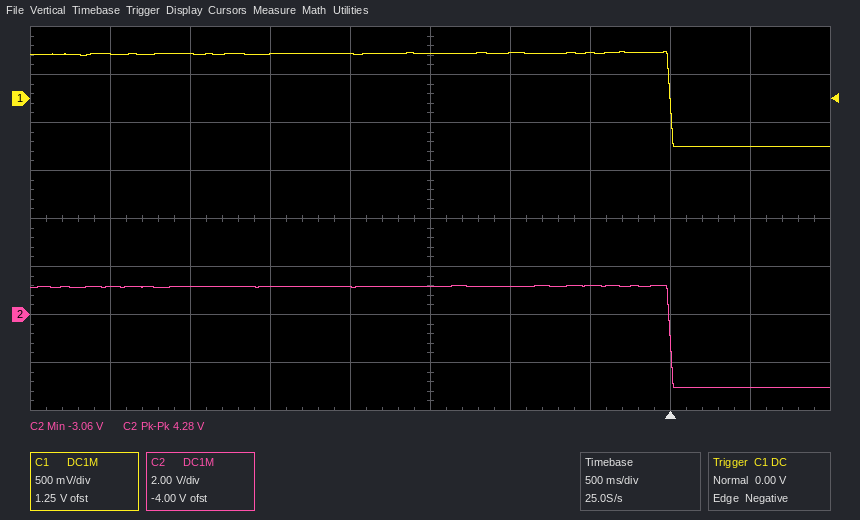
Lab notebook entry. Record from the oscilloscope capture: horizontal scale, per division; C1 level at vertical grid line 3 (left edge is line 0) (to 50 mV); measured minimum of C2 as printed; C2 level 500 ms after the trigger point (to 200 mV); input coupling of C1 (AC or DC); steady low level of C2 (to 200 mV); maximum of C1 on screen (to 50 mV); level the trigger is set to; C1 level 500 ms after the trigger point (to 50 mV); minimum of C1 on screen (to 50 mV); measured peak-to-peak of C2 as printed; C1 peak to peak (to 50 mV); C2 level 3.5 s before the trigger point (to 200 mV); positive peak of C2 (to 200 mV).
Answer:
500 ms
450 mV
-3.06 V
-3.0 V
DC
-3.0 V
500 mV
0.00 V
-500 mV
-500 mV
4.28 V
1.00 V
1.2 V
1.2 V
